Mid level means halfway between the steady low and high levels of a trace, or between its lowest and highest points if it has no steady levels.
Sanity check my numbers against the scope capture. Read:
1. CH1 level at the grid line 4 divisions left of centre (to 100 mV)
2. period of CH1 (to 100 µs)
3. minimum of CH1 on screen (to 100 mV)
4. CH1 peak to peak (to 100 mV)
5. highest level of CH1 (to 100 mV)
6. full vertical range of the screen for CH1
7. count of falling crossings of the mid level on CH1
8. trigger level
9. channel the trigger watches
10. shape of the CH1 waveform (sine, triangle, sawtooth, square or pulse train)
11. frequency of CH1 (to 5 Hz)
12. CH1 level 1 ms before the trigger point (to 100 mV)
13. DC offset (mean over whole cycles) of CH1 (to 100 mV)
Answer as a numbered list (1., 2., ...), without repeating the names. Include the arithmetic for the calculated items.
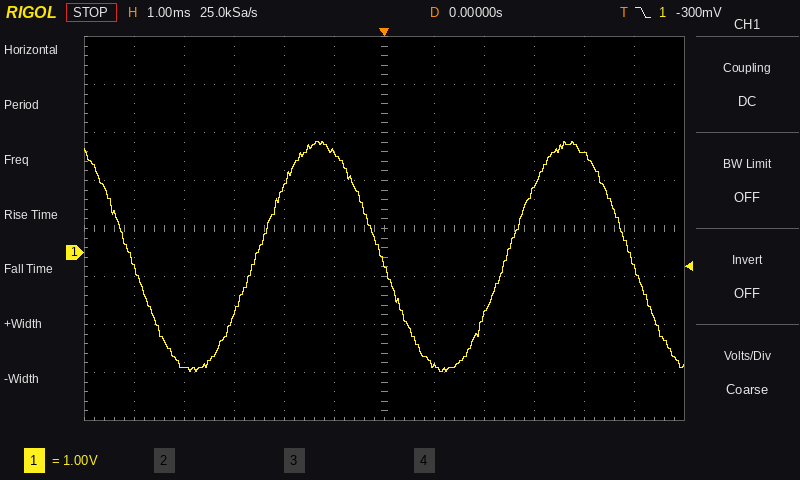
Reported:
1. -2.4 V
2. 5.0 ms
3. -2.5 V
4. 2.3 V − (-2.5 V) = 4.8 V
5. 2.3 V
6. 8 V
7. 3
8. -300 mV
9. CH1
10. sine
11. 1 / 5.0 ms ≈ 200 Hz
12. 2.1 V
13. (2.3 V + (-2.5 V)) / 2 ≈ -100 mV
